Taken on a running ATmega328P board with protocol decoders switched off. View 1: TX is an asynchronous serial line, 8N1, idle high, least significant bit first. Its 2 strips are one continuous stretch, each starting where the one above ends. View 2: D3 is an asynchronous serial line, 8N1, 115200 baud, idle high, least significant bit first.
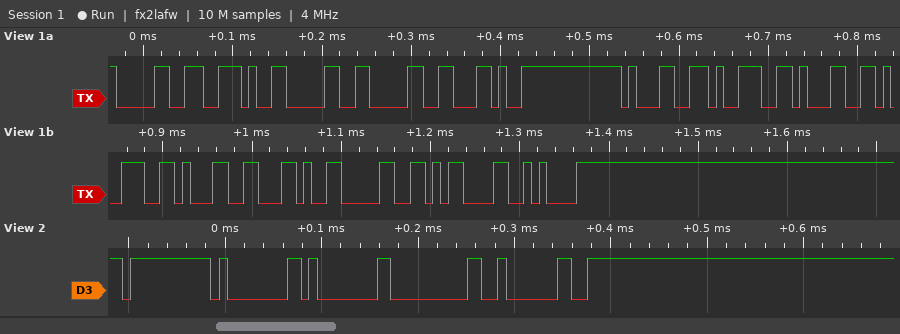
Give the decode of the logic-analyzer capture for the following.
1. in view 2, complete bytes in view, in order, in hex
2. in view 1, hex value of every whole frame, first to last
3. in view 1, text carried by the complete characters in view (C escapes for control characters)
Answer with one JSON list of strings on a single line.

["0xFF 0x01 0x01 0x00 0x02 0xFE", "30 2E 30 30 2C 31 39 31 39 31 2C 30 0D 0A", "\"0.00,19191,0\\r\\n\""]
